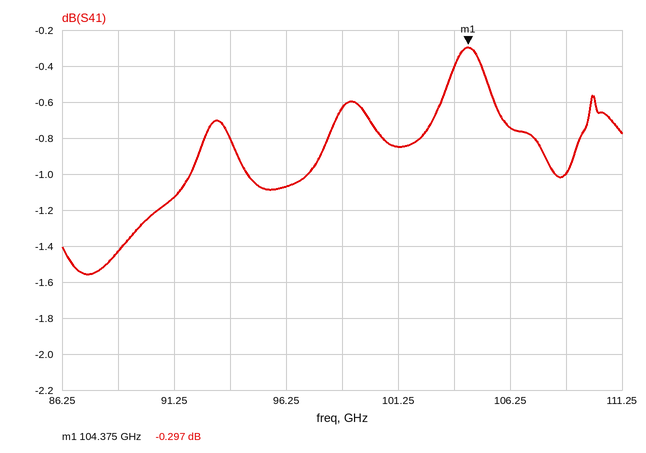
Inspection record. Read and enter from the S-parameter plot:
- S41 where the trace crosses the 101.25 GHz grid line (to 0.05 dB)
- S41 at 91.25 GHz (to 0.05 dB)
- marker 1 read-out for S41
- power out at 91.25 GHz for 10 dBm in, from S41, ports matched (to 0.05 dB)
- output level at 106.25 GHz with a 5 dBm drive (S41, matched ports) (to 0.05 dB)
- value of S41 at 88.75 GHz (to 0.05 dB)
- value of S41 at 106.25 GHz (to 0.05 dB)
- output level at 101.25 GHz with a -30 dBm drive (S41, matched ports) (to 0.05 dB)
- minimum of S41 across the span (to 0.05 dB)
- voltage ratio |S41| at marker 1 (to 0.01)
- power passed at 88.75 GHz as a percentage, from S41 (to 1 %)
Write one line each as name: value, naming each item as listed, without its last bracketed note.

S41 where the trace crosses the 101.25 GHz grid line: -0.85 dB
S41 at 91.25 GHz: -1.15 dB
marker 1 read-out for S41: -0.297 dB
power out at 91.25 GHz for 10 dBm in, from S41, ports matched: 8.85 dBm
output level at 106.25 GHz with a 5 dBm drive (S41, matched ports): 4.25 dBm
value of S41 at 88.75 GHz: -1.45 dB
value of S41 at 106.25 GHz: -0.75 dB
output level at 101.25 GHz with a -30 dBm drive (S41, matched ports): -30.85 dBm
minimum of S41 across the span: -1.55 dB
voltage ratio |S41| at marker 1: 0.97
power passed at 88.75 GHz as a percentage, from S41: 72 %
